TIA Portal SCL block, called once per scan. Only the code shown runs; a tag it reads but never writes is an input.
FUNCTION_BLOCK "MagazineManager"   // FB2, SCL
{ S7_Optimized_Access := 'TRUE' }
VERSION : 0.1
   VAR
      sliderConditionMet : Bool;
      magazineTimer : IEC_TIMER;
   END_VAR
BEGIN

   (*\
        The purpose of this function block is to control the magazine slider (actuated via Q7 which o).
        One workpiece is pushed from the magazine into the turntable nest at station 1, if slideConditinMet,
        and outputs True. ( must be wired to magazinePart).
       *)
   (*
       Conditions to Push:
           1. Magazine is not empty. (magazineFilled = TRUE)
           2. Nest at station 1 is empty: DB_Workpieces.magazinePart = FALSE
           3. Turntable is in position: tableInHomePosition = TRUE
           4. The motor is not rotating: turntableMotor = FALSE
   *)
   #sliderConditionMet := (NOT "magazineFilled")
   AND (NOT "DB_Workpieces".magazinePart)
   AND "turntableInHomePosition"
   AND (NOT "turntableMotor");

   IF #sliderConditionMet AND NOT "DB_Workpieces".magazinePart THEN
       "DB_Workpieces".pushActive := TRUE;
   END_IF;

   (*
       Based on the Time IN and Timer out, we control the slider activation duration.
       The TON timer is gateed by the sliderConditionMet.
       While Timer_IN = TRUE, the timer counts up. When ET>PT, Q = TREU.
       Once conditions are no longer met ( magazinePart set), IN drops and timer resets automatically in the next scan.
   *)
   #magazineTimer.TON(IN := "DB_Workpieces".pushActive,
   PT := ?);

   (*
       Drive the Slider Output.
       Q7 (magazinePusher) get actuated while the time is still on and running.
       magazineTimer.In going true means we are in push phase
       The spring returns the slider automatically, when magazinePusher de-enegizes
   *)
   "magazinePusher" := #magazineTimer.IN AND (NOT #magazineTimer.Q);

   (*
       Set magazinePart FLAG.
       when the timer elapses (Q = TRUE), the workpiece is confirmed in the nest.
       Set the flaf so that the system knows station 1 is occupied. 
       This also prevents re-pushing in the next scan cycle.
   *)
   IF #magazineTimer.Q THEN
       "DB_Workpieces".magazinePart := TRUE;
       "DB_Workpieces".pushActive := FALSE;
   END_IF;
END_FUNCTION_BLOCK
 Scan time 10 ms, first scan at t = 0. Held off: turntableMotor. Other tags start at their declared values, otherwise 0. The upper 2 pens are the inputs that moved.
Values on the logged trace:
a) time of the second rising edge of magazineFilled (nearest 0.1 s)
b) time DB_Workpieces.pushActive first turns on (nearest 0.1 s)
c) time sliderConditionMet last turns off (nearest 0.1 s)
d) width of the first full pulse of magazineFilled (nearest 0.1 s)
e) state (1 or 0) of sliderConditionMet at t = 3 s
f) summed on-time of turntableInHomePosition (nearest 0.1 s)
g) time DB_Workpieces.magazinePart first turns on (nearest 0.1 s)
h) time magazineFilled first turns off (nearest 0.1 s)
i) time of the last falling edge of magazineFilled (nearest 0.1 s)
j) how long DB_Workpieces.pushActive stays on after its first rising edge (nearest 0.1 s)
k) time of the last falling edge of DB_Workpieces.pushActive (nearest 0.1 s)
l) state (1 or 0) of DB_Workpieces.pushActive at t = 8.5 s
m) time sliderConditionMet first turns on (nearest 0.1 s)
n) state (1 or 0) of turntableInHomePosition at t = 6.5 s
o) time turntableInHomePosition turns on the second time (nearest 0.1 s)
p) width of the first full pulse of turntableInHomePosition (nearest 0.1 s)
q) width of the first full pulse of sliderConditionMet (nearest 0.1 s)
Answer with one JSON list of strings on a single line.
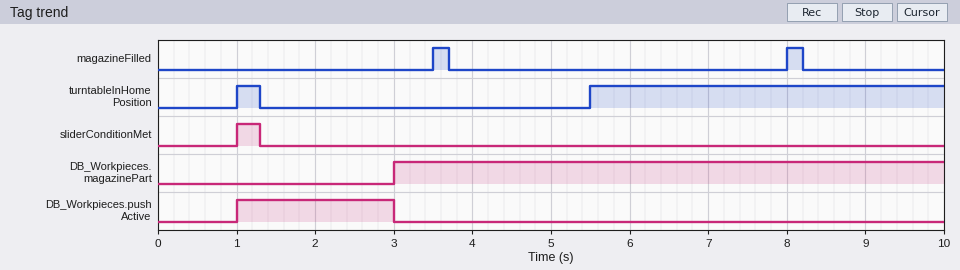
["8.0 s", "1.0 s", "1.3 s", "0.2 s", "0", "4.8 s", "3.0 s", "3.7 s", "8.2 s", "2.0 s", "3.0 s", "0", "1.0 s", "1", "5.5 s", "0.3 s", "0.3 s"]
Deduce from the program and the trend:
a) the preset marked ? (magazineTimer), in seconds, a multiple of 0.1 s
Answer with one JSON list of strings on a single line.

["2.0 s"]
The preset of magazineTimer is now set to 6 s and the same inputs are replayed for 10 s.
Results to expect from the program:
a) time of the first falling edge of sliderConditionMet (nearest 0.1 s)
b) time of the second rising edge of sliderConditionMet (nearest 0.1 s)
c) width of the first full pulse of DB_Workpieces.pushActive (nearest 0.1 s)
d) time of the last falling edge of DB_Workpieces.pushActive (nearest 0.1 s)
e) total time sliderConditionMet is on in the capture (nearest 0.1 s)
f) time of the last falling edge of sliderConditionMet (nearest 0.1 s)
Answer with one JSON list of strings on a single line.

["1.3 s", "5.5 s", "6.0 s", "7.0 s", "1.8 s", "7.0 s"]
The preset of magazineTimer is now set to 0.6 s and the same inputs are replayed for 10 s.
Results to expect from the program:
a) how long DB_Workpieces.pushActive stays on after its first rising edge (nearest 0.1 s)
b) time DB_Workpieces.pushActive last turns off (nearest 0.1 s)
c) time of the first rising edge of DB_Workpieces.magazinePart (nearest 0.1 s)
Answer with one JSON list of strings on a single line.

["0.6 s", "1.6 s", "1.6 s"]
